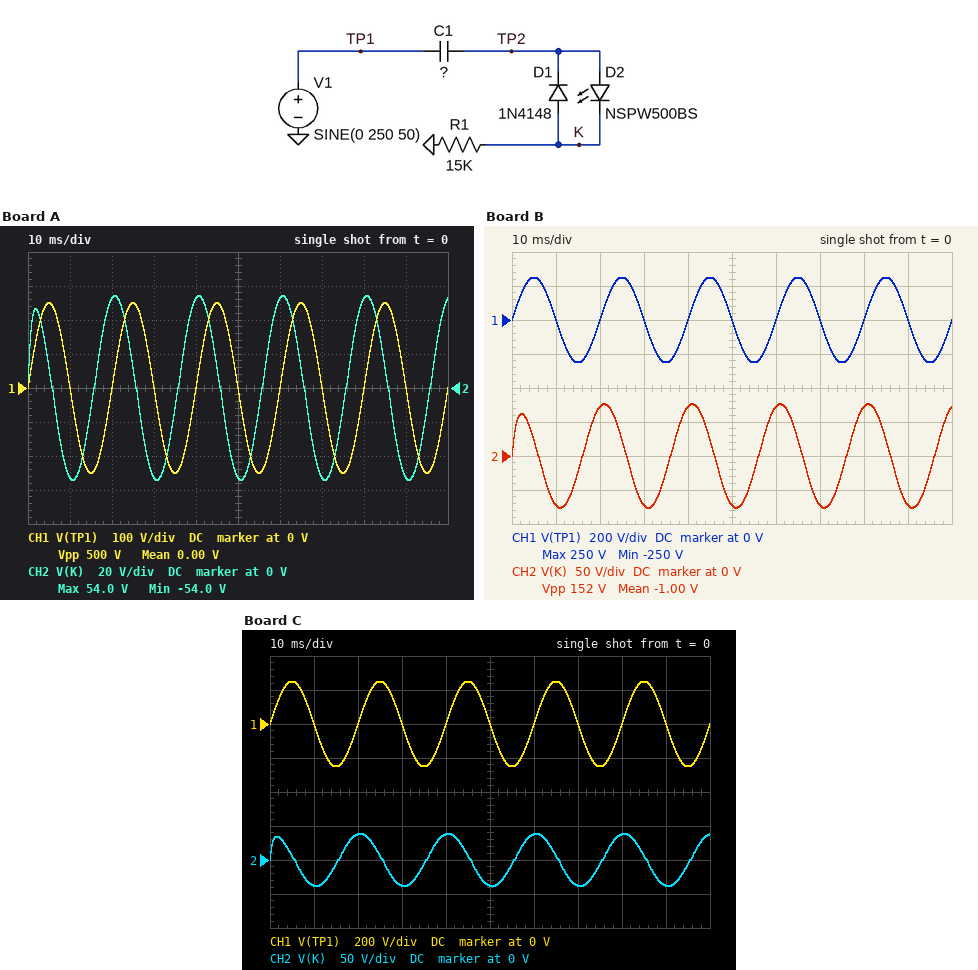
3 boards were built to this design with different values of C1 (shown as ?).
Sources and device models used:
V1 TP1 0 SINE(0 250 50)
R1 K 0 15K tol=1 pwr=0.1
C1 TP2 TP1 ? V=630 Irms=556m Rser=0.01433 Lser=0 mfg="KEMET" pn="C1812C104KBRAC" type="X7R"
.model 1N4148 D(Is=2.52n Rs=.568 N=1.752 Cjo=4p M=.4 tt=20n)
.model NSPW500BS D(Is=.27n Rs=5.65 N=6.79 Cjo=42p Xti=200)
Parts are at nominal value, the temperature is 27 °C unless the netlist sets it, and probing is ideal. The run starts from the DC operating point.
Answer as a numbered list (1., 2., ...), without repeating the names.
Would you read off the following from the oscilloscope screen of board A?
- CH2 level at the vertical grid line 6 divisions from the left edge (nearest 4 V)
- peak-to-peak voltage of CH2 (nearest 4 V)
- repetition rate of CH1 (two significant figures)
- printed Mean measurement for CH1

1. 52 V
2. 108 V
3. 50 Hz
4. 0.00 V
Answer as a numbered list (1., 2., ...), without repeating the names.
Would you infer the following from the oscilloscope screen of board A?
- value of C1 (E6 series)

1. 47 nF
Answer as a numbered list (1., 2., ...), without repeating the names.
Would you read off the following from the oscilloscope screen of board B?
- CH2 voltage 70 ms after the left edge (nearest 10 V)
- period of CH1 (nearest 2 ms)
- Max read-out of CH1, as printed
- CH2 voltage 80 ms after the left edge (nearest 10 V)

1. -70 V
2. 20 ms
3. 250 V
4. 70 V
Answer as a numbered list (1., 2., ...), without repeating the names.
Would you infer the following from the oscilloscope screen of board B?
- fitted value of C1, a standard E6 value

1. 68 nF
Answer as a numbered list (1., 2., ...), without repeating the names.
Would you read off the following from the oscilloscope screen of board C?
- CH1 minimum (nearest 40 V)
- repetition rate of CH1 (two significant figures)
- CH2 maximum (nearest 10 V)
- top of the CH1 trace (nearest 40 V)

1. -240 V
2. 50 Hz
3. 40 V
4. 240 V
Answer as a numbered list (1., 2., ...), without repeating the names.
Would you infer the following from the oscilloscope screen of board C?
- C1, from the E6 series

1. 33 nF
